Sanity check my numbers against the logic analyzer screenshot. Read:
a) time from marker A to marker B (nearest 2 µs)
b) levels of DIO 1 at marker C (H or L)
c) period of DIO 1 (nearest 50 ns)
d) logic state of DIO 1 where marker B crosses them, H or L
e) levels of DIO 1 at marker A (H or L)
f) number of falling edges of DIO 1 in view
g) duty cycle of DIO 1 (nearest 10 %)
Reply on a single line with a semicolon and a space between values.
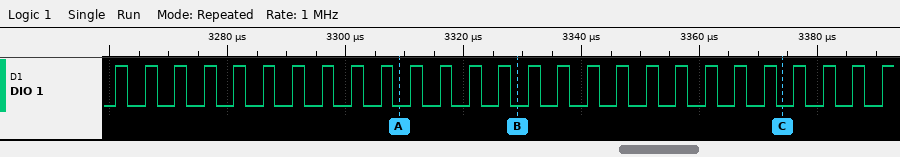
20 µs; DIO 1=L; 5000 ns; DIO 1=L; DIO 1=L; 26; 40 %
